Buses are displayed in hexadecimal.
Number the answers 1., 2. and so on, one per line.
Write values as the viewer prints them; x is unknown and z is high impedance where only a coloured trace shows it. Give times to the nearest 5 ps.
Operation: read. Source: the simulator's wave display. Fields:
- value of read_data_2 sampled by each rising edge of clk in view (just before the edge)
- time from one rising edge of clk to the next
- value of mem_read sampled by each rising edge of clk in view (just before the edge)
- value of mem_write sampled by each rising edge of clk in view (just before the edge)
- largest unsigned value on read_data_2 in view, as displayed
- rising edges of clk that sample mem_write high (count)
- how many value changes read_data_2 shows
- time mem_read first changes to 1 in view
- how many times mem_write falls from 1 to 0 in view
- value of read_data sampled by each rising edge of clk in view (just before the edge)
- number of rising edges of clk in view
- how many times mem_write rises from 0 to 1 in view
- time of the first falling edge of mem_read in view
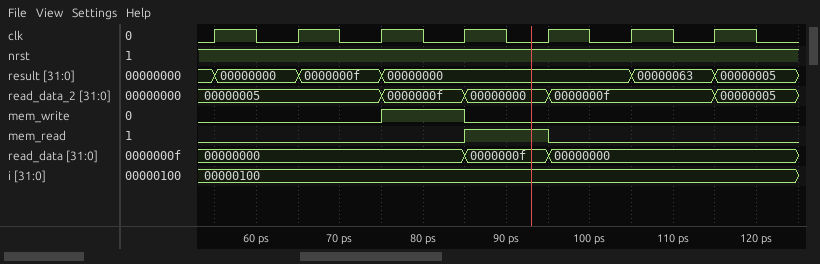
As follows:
1. 00000005, 00000005, 00000005, 0000000f, 00000000, 0000000f, 0000000f
2. 10 ps
3. 0 0 0 0 1 0 0
4. 0 0 0 1 0 0 0
5. 0000000f
6. 1
7. 4
8. 85 ps
9. 1
10. 00000000, 00000000, 00000000, 00000000, 0000000f, 00000000, 00000000
11. 7
12. 1
13. 95 ps
